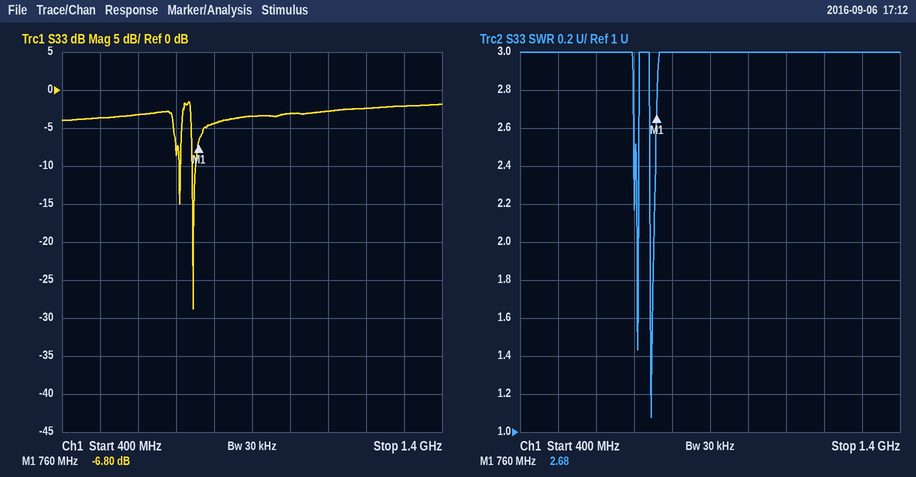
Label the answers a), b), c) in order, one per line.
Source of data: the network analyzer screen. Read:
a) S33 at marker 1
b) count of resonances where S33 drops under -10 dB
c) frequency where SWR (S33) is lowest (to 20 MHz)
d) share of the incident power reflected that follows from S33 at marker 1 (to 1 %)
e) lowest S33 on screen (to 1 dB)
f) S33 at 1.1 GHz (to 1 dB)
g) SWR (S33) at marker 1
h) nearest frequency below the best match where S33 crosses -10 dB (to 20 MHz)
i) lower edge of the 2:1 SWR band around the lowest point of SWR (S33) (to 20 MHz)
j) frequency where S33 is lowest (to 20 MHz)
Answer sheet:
a) -6.80 dB
b) 2
c) 740 MHz
d) 21 %
e) -29 dB
f) -3 dB
g) 2.68
h) 740 MHz
i) 740 MHz
j) 740 MHz
